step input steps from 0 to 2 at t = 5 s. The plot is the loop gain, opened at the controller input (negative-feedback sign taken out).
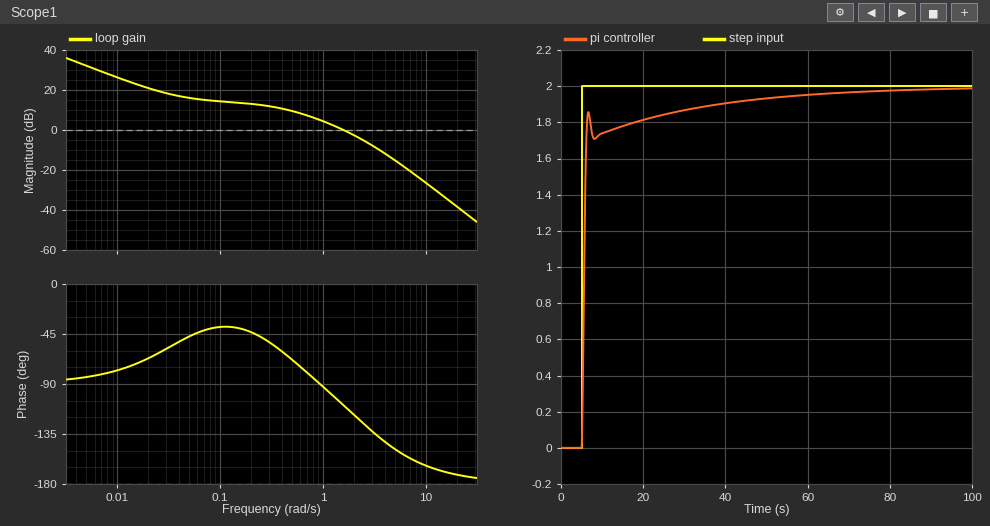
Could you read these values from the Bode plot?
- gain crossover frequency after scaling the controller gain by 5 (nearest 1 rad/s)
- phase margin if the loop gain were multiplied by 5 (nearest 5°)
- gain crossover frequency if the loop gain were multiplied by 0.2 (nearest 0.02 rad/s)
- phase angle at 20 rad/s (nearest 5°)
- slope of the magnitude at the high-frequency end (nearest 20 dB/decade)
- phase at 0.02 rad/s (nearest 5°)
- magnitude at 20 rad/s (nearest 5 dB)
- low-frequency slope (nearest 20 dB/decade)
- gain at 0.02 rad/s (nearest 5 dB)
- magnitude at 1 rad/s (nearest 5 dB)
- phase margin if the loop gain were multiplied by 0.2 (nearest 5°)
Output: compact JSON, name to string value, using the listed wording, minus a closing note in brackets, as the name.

{"gain crossover frequency after scaling the controller gain by 5": "5 rad/s", "phase margin if the loop gain were multiplied by 5": "35°", "gain crossover frequency if the loop gain were multiplied by 0.2": "0.12 rad/s", "phase angle at 20 rad/s": "-170°", "slope of the magnitude at the high-frequency end": "-40 dB/decade", "phase at 0.02 rad/s": "-65°", "magnitude at 20 rad/s": "-40 dB", "low-frequency slope": "-20 dB/decade", "gain at 0.02 rad/s": "20 dB", "magnitude at 1 rad/s": "5 dB", "phase margin if the loop gain were multiplied by 0.2": "140°"}
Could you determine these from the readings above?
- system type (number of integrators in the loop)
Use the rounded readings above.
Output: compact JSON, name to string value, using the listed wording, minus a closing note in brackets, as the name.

{"system type": "1"}
